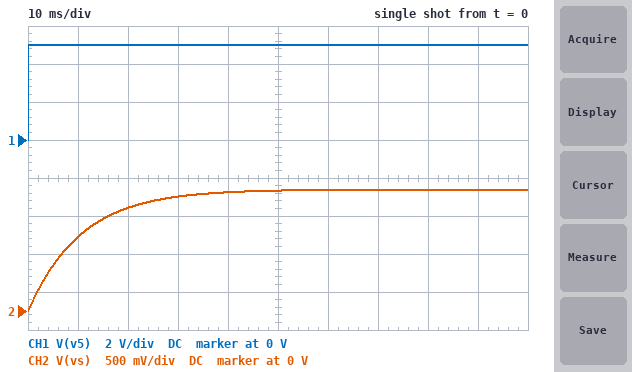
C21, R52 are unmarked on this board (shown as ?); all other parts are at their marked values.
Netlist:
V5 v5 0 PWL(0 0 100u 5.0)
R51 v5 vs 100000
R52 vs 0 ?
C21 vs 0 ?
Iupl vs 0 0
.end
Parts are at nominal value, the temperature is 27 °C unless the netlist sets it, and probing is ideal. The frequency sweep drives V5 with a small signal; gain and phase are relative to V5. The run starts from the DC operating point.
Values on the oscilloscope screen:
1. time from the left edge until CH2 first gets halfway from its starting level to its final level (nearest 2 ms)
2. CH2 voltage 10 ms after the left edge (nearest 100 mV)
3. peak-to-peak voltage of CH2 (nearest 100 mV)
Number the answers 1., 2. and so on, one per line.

1. 8 ms
2. 1.0 V
3. 1.6 V
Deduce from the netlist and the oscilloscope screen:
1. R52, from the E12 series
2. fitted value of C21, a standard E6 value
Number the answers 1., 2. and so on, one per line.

1. 47 kΩ
2. 330 nF
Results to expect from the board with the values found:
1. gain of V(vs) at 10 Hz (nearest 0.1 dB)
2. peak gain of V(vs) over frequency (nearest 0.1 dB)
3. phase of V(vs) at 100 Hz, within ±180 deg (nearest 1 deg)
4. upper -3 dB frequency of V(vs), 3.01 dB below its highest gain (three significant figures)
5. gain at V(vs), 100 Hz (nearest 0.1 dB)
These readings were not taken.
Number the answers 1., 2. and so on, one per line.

1. -11.5 dB
2. -9.9 dB
3. -81 deg
4. 15.1 Hz
5. -26.4 dB
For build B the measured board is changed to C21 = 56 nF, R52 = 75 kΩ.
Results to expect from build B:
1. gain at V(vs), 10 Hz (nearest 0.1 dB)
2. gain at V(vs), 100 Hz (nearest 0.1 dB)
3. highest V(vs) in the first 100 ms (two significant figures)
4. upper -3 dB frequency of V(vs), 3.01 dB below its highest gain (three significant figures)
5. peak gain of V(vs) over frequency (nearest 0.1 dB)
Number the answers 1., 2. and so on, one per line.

1. -7.5 dB
2. -12.5 dB
3. 2.1 V
4. 66.3 Hz
5. -7.4 dB
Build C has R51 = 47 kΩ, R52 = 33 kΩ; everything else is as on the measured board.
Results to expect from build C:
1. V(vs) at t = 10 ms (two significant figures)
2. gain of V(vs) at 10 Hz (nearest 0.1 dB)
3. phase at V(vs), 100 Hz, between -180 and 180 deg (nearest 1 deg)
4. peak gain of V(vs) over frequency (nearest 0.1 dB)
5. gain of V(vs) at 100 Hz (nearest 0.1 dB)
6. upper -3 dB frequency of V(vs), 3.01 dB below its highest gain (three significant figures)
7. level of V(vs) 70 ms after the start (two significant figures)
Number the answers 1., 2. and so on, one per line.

1. 1.6 V
2. -8.3 dB
3. -76 deg
4. -7.7 dB
5. -20.0 dB
6. 24.9 Hz
7. 2.1 V
